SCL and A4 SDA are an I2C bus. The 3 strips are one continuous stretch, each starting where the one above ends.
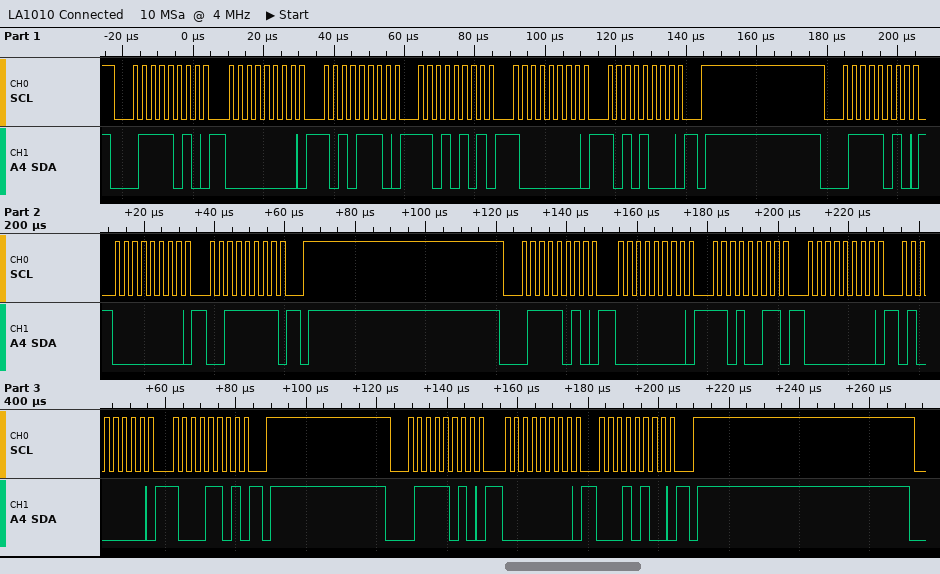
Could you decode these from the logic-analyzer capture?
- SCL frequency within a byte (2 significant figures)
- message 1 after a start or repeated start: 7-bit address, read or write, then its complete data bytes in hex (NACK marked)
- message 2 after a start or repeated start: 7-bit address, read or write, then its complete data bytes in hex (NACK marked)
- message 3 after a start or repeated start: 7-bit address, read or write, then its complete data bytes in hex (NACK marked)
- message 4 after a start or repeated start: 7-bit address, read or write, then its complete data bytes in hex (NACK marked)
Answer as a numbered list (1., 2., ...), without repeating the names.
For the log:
1. 400 kHz
2. 0x3D write: 00 AE D5 80 A8
3. 0x3D write: 00 3F
4. 0x3D write: 00 D3 00 40 8D
5. 0x3D write: 00 14
